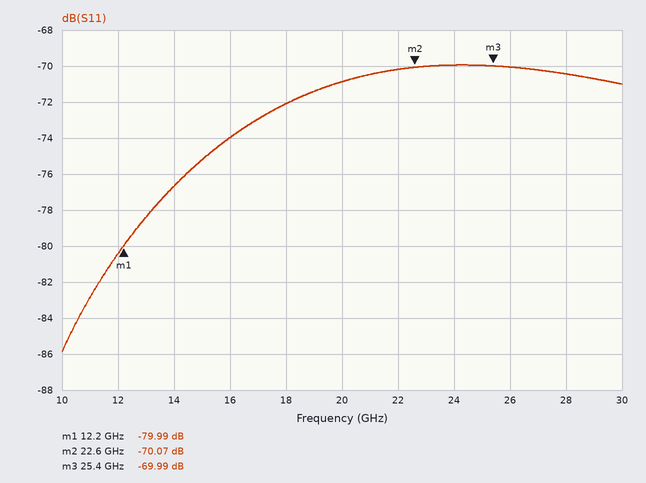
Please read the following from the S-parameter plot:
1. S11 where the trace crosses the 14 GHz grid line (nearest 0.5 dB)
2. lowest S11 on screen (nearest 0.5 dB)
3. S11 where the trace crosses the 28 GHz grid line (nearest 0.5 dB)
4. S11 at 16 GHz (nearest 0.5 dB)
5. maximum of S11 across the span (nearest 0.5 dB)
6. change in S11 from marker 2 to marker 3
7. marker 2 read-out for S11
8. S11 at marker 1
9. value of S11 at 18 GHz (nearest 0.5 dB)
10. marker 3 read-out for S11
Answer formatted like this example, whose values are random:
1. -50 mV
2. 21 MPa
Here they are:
1. -76.5 dB
2. -86.0 dB
3. -70.5 dB
4. -74.0 dB
5. -70.0 dB
6. 0.08 dB
7. -70.07 dB
8. -79.99 dB
9. -72.0 dB
10. -69.99 dB
